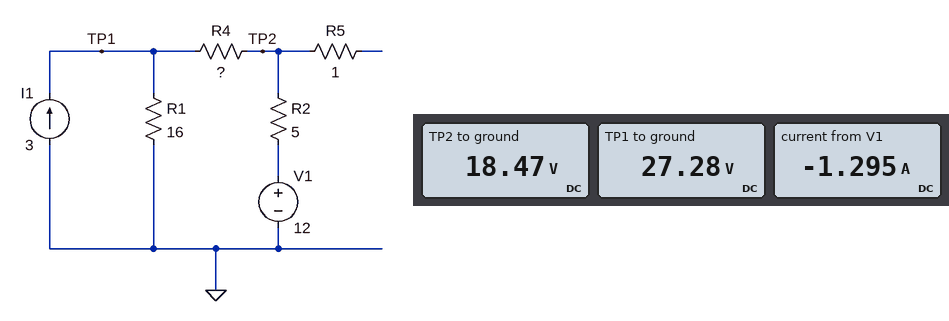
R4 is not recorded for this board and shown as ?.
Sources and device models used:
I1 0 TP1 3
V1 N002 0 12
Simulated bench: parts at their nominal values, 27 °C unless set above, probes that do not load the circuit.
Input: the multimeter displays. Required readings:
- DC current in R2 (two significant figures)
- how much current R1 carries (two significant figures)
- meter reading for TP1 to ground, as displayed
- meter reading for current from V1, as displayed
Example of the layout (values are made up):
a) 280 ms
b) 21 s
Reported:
a) 1.3 A
b) 1.7 A
c) 27.28 V
d) -1.295 A
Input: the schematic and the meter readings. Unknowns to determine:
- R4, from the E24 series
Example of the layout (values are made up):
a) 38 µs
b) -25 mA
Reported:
a) 6.8 Ω
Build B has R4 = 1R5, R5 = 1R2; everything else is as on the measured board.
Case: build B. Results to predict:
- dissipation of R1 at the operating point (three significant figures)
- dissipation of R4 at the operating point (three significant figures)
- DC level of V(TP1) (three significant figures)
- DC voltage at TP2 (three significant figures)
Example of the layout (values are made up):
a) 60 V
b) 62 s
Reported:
a) 31.4 W
b) 3.84 W
c) 22.4 V
d) 20.0 V
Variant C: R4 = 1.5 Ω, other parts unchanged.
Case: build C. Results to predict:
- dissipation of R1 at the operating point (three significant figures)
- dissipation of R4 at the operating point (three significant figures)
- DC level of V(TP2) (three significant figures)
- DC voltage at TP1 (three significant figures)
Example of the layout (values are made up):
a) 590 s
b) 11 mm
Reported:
a) 31.4 W
b) 3.84 W
c) 20.0 V
d) 22.4 V
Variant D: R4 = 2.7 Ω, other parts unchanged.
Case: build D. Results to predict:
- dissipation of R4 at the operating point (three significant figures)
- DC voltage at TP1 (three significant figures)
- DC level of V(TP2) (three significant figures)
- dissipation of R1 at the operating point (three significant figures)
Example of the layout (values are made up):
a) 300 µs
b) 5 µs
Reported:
a) 6.23 W
b) 23.7 V
c) 19.6 V
d) 35.1 W
